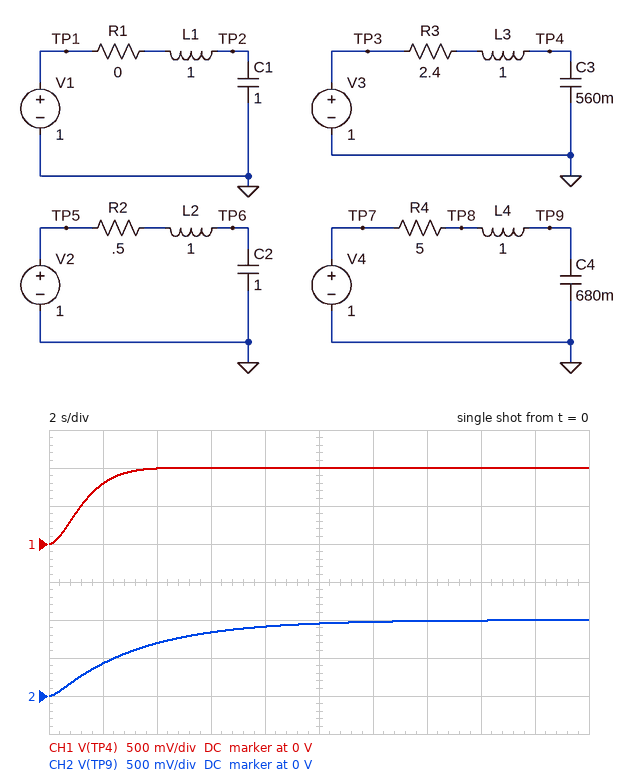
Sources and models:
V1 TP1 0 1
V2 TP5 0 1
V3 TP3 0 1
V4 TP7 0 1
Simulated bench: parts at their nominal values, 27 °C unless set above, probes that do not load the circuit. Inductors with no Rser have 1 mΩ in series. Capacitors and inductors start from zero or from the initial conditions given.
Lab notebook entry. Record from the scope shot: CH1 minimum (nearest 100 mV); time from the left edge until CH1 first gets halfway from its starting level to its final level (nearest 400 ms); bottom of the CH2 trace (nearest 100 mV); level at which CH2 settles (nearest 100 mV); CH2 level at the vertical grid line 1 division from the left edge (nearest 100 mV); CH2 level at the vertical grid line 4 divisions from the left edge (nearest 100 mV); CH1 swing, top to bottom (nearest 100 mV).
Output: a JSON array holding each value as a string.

["0 V", "1.2 s", "0 V", "1.0 V", "400 mV", "900 mV", "1.0 V"]
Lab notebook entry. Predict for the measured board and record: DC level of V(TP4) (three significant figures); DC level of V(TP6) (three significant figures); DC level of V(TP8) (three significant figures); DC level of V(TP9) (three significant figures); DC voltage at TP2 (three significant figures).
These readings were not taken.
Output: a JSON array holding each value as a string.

["1.00 V", "1.00 V", "1.00 V", "1.00 V", "1.00 V"]
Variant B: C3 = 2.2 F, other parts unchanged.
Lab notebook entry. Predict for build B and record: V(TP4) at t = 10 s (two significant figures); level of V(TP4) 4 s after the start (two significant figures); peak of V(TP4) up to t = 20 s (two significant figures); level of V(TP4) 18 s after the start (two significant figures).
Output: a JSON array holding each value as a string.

["860 mV", "520 mV", "980 mV", "970 mV"]
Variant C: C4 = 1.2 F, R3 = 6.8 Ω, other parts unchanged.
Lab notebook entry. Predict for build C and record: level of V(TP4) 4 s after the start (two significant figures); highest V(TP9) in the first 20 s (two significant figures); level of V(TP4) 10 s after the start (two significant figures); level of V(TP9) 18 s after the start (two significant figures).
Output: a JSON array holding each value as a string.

["650 mV", "970 mV", "930 mV", "950 mV"]
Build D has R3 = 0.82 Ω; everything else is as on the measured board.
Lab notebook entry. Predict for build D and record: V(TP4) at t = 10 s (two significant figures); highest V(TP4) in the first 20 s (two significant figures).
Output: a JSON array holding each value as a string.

["980 mV", "1.4 V"]
